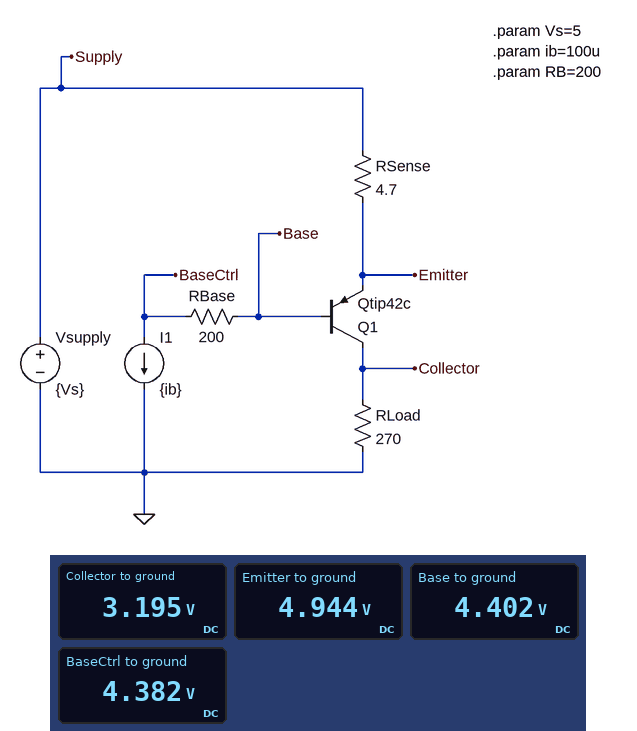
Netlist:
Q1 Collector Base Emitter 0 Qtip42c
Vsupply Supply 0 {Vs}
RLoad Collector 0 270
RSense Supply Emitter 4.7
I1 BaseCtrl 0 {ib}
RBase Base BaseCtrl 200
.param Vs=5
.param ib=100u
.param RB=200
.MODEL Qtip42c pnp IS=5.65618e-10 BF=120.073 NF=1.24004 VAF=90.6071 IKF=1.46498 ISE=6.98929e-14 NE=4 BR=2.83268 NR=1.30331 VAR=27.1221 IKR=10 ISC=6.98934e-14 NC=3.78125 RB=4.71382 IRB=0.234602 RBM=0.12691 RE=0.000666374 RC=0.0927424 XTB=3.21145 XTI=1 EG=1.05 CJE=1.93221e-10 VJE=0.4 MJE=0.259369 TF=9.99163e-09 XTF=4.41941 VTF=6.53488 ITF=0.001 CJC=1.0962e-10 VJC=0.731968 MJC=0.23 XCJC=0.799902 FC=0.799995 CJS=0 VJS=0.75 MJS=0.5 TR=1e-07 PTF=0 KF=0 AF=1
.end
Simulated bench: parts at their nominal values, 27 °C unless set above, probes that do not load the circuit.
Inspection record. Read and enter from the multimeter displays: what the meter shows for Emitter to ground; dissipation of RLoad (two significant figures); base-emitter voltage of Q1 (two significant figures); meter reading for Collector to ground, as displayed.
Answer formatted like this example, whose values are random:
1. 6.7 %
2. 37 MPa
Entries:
1. 4.944 V
2. 38 mW
3. -540 mV
4. 3.195 V
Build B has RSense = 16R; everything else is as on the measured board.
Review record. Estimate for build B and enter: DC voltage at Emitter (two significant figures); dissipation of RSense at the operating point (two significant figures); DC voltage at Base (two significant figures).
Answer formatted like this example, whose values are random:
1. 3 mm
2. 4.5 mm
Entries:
1. 4.8 V
2. 2.3 mW
3. 4.3 V
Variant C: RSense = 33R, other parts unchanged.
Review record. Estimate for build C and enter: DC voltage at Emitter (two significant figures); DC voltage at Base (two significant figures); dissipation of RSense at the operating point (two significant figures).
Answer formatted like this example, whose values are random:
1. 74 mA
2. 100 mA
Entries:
1. 4.6 V
2. 4.1 V
3. 4.7 mW
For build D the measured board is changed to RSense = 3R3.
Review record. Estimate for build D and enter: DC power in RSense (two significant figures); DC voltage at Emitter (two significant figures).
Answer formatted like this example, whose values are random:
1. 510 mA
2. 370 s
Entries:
1. 470 µW
2. 5.0 V
